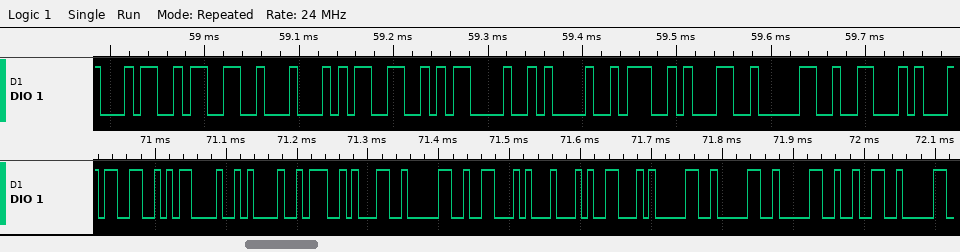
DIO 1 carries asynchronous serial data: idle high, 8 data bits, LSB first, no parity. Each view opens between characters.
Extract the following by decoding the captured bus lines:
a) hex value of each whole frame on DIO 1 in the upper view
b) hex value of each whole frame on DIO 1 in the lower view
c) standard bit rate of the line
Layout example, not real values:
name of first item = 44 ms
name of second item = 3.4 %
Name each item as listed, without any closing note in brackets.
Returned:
hex value of each whole frame on DIO 1 in the upper view = 34, 33, 44, 33, 0D, 0A, 3A, 31, 30, 46
hex value of each whole frame on DIO 1 in the lower view = 33, 0D, 0A, 3A, 31, 30, 46, 44, 46, 30, 30, 30, 32
standard bit rate of the line = 115200 baud
